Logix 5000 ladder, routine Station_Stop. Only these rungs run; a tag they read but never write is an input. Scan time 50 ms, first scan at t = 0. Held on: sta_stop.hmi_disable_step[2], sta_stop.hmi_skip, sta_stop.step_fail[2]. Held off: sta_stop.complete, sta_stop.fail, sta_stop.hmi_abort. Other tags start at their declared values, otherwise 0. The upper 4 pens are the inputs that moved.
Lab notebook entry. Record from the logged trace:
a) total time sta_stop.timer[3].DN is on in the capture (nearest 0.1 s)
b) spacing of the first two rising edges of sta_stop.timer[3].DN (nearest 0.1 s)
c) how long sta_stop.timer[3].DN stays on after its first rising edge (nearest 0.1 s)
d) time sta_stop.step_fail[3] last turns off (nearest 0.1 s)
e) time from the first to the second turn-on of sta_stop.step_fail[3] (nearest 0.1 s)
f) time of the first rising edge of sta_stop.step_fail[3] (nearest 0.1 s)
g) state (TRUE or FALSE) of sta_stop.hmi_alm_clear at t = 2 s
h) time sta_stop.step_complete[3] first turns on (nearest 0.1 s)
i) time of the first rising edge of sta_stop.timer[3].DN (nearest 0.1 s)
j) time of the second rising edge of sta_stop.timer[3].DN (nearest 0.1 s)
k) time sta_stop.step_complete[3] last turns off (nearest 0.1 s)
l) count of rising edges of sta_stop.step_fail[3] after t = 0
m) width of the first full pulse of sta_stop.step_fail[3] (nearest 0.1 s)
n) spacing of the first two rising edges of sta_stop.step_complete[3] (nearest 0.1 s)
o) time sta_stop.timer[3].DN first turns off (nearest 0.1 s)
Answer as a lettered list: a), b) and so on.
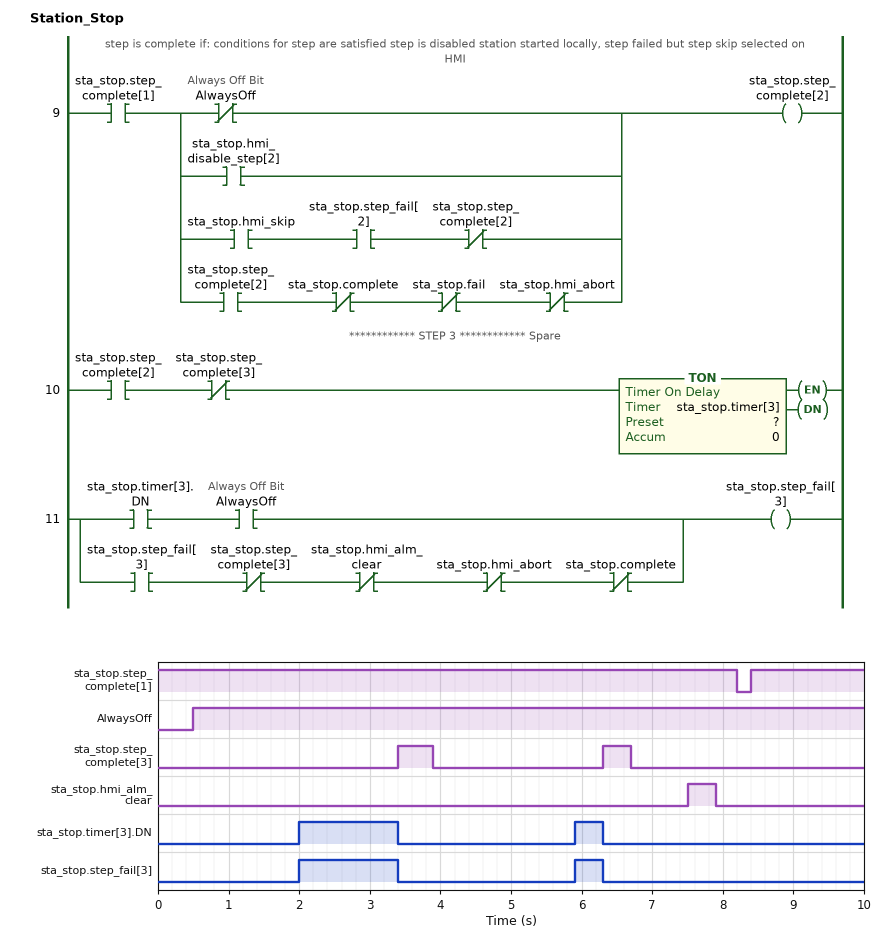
a) 1.8 s
b) 3.9 s
c) 1.4 s
d) 6.3 s
e) 3.9 s
f) 2.0 s
g) FALSE
h) 3.4 s
i) 2.0 s
j) 5.9 s
k) 6.7 s
l) 2
m) 1.4 s
n) 2.9 s
o) 3.4 s
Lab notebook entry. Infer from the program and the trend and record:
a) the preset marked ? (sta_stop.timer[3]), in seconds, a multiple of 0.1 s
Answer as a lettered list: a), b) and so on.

a) 2.0 s
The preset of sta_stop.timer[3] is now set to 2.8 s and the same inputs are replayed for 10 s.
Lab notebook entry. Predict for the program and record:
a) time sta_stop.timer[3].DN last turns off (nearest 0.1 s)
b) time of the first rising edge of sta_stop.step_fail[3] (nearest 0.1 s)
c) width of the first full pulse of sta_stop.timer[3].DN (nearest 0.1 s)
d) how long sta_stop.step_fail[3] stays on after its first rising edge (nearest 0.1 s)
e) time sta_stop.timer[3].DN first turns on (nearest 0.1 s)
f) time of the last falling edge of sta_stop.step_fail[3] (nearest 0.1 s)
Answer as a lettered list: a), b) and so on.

a) 3.4 s
b) 2.8 s
c) 0.6 s
d) 0.6 s
e) 2.8 s
f) 3.4 s
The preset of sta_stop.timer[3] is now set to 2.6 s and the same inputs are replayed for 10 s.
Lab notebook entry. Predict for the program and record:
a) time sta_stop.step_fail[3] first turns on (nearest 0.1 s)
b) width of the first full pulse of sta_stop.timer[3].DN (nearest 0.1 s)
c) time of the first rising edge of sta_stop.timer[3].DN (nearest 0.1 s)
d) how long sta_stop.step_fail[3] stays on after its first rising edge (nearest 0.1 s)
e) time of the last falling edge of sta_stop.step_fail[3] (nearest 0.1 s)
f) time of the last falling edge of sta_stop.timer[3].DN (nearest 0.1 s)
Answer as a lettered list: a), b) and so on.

a) 2.6 s
b) 0.8 s
c) 2.6 s
d) 0.8 s
e) 3.4 s
f) 3.4 s
